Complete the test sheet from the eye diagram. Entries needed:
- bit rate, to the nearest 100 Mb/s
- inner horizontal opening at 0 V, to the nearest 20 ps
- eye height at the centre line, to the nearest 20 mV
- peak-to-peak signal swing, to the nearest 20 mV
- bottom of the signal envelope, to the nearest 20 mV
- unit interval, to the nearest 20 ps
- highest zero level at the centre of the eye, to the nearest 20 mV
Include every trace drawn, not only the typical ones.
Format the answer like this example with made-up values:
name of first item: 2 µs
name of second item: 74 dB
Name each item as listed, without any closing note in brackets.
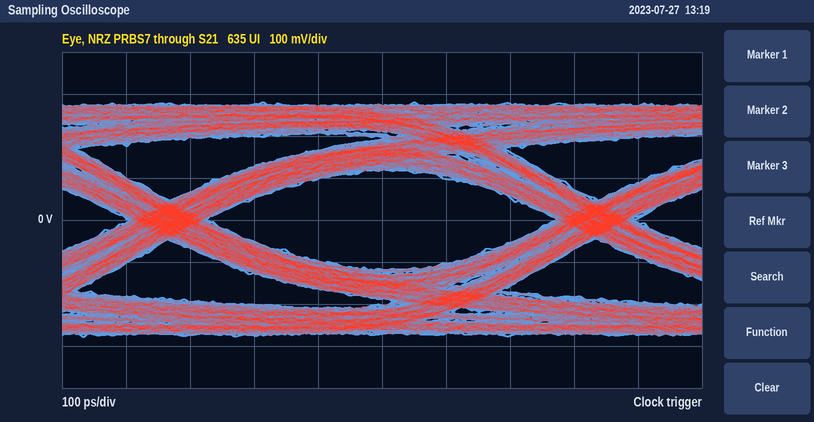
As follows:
bit rate, to the nearest 100 Mb/s: 1.5 Gb/s
inner horizontal opening at 0 V, to the nearest 20 ps: 540 ps
eye height at the centre line, to the nearest 20 mV: 240 mV
peak-to-peak signal swing, to the nearest 20 mV: 560 mV
bottom of the signal envelope, to the nearest 20 mV: -280 mV
unit interval, to the nearest 20 ps: 660 ps
highest zero level at the centre of the eye, to the nearest 20 mV: -120 mV
